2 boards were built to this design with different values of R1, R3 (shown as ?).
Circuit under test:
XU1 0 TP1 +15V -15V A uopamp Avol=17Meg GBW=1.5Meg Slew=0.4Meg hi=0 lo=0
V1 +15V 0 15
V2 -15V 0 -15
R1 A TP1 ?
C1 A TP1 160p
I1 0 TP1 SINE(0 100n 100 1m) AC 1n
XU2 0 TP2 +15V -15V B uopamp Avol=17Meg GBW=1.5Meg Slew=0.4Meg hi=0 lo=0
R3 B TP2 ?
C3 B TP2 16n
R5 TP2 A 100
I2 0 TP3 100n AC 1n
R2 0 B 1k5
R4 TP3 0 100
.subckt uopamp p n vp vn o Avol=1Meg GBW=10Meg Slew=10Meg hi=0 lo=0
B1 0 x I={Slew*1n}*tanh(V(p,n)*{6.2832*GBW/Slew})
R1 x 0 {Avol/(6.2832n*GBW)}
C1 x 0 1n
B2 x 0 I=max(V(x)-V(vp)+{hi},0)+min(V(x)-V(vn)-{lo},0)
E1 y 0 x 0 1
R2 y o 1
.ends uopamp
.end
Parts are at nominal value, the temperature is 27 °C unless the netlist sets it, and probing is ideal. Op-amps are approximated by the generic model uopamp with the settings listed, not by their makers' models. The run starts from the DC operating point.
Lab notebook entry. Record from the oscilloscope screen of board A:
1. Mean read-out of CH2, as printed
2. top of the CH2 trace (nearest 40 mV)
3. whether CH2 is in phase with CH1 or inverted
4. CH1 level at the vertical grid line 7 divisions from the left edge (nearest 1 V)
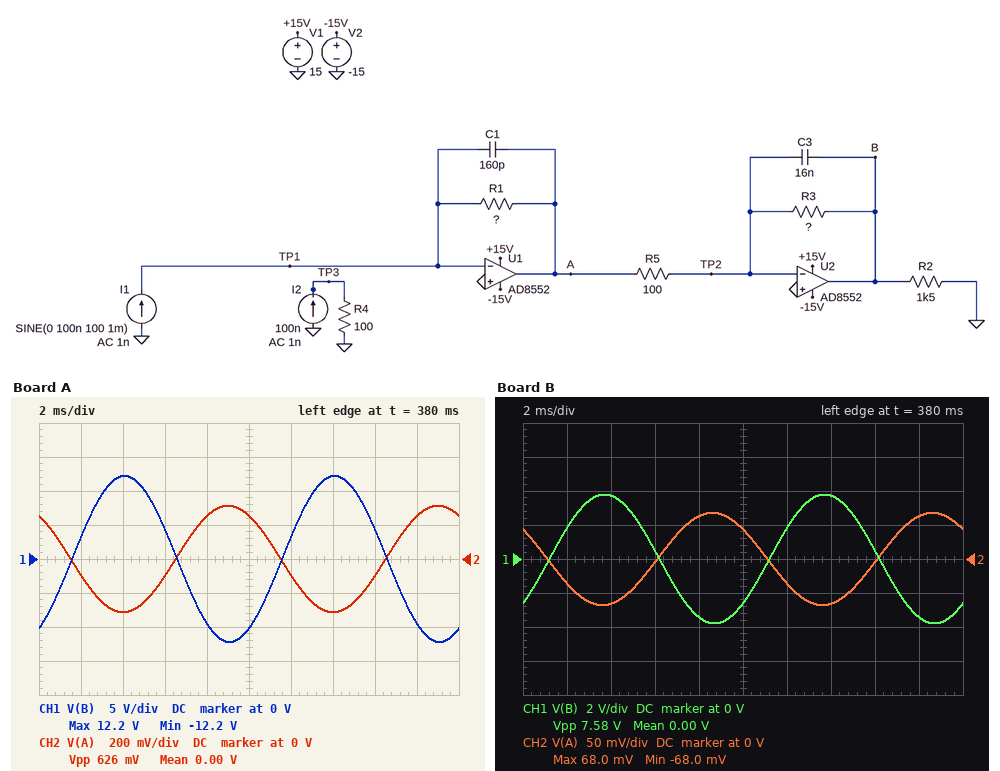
0.00 V
320 mV
inverted
12 V
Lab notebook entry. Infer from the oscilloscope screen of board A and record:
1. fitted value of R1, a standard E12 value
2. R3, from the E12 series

3.3 MΩ
3.9 kΩ
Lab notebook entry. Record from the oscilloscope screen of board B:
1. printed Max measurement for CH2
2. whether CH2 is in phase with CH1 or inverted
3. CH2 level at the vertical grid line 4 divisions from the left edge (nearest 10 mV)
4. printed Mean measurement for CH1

68.0 mV
inverted
60 mV
0.00 V
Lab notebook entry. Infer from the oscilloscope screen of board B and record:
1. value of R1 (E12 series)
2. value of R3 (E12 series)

680 kΩ
5.6 kΩ
